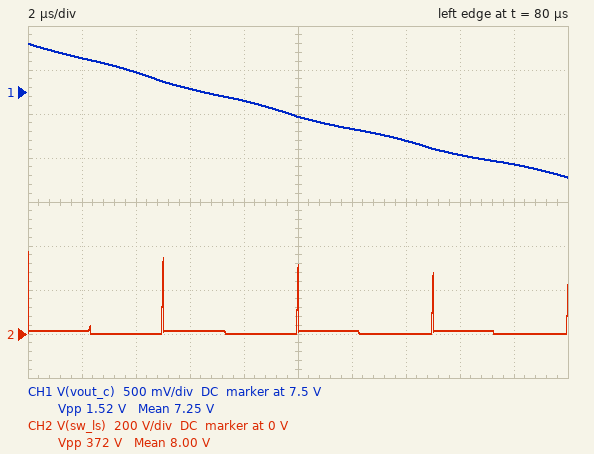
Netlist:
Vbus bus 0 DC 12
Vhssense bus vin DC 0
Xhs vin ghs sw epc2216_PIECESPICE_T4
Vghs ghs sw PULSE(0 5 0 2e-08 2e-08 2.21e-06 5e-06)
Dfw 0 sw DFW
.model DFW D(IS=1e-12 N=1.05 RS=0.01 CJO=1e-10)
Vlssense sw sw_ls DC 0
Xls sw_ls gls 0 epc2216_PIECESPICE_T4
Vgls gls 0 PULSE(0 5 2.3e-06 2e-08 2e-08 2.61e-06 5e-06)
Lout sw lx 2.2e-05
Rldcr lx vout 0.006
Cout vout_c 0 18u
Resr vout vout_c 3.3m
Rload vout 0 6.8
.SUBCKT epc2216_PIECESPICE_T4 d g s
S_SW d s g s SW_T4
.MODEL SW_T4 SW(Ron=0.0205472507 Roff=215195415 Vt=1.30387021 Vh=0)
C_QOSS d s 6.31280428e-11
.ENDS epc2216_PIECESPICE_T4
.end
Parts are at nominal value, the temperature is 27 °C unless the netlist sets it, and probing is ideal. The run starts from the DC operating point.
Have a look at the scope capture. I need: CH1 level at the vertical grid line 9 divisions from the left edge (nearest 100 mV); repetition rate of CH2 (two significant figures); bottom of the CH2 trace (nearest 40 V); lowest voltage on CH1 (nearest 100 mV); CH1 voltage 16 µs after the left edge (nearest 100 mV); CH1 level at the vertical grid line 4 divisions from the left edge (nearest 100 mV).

6.7 V
200 kHz
0 V
6.5 V
6.8 V
7.4 V
